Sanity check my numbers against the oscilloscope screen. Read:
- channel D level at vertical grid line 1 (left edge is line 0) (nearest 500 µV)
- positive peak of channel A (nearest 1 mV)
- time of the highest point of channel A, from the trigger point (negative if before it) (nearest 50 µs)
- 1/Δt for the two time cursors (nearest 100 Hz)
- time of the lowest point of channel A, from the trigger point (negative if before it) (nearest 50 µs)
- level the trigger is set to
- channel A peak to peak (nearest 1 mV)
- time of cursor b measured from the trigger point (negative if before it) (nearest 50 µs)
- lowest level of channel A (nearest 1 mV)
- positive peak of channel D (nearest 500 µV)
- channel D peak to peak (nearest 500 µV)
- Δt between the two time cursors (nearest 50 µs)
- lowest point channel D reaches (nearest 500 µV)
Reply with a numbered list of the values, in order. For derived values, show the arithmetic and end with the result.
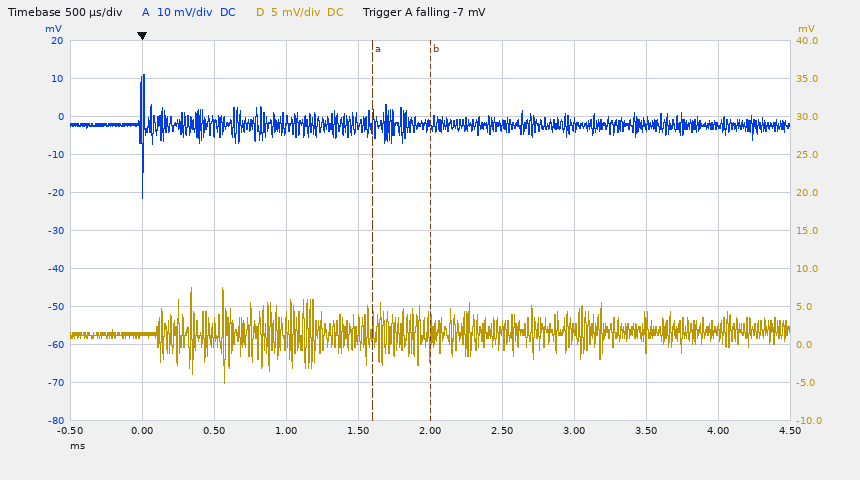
1. 1.0 mV
2. 11 mV
3. 0 µs
4. 1 / 400 µs ≈ 2.5 kHz
5. 0 µs
6. -7 mV
7. 11 mV − (-22 mV) = 33 mV
8. +2.00 ms
9. -22 mV
10. 7.5 mV
11. 7.5 mV − (-5.0 mV) = 12.5 mV
12. 400 µs
13. -5.0 mV
